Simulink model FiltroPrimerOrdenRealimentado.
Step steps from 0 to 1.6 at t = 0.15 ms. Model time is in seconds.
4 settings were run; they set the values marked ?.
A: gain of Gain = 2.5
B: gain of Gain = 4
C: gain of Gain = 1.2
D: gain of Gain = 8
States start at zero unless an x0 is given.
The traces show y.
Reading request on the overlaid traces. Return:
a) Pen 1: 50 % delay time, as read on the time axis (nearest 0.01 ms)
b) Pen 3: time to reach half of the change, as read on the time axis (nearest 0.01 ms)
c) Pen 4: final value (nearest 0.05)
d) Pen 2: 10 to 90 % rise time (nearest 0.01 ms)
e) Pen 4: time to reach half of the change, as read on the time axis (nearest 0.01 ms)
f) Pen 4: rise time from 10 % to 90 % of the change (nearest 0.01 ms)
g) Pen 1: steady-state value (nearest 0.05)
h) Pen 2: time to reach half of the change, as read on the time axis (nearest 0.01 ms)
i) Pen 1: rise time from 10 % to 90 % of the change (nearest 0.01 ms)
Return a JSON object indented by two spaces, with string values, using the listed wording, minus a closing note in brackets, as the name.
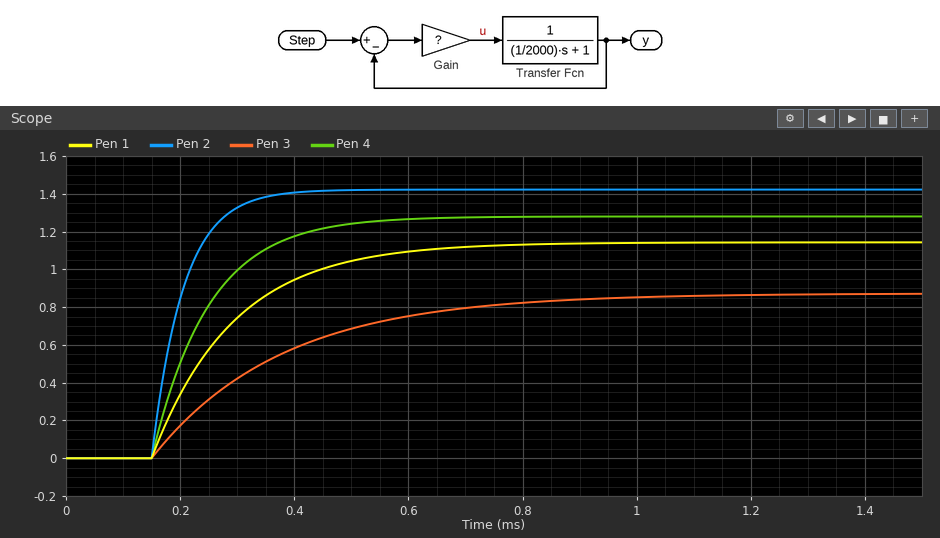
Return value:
{
  "Pen 1: 50 % delay time, as read on the time axis": "0.25 ms",
  "Pen 3: time to reach half of the change, as read on the time axis": "0.31 ms",
  "Pen 4: final value": "1.30",
  "Pen 2: 10 to 90 % rise time": "0.12 ms",
  "Pen 4: time to reach half of the change, as read on the time axis": "0.22 ms",
  "Pen 4: rise time from 10 % to 90 % of the change": "0.22 ms",
  "Pen 1: steady-state value": "1.15",
  "Pen 2: time to reach half of the change, as read on the time axis": "0.19 ms",
  "Pen 1: rise time from 10 % to 90 % of the change": "0.31 ms"
}
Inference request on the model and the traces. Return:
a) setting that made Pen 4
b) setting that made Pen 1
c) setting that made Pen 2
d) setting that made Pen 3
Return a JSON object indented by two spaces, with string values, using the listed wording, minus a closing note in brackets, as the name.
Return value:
{
  "setting that made Pen 4": "B",
  "setting that made Pen 1": "A",
  "setting that made Pen 2": "D",
  "setting that made Pen 3": "C"
}
